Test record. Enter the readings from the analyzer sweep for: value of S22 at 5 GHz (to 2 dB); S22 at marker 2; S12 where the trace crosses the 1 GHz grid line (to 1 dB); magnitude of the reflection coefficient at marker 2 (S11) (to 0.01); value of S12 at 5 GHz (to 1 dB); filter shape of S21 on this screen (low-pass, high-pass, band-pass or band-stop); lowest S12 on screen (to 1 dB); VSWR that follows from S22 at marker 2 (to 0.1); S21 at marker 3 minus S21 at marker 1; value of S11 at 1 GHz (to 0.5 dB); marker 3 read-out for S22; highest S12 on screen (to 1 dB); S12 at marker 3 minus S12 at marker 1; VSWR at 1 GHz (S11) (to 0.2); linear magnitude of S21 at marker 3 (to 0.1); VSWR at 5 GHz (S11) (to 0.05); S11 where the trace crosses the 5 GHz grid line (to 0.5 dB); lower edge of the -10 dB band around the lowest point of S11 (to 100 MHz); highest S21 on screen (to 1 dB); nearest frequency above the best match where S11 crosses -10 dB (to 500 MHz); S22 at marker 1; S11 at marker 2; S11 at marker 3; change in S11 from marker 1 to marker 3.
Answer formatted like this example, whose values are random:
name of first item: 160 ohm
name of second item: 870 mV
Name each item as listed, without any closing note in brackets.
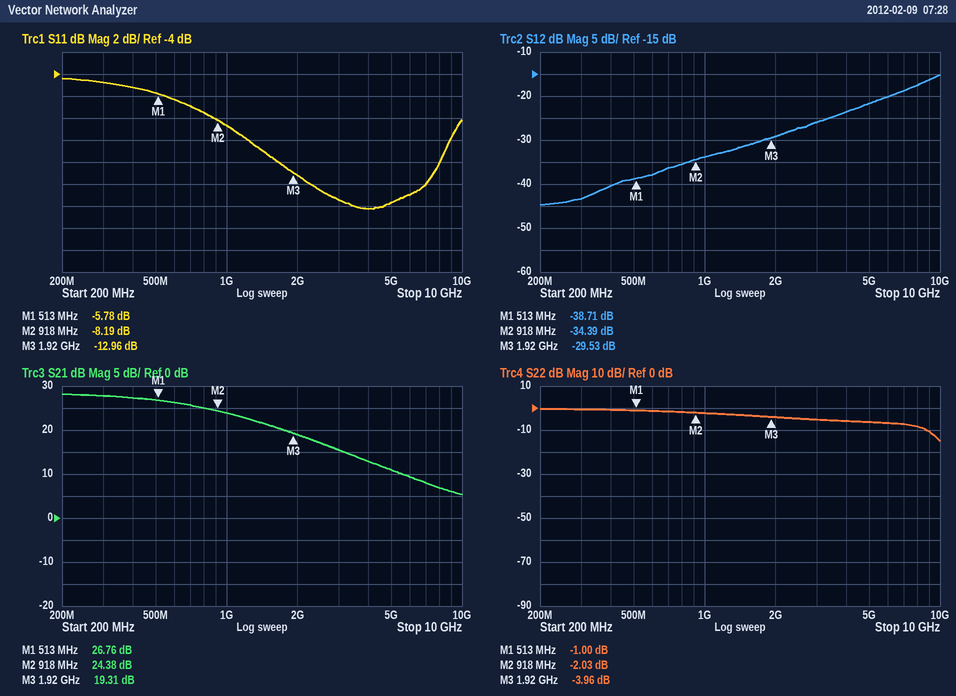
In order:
value of S22 at 5 GHz: -6 dB
S22 at marker 2: -2.03 dB
S12 where the trace crosses the 1 GHz grid line: -34 dB
magnitude of the reflection coefficient at marker 2 (S11): 0.39
value of S12 at 5 GHz: -22 dB
filter shape of S21 on this screen: low-pass
lowest S12 on screen: -45 dB
VSWR that follows from S22 at marker 2: 8.6
S21 at marker 3 minus S21 at marker 1: -7.45 dB
value of S11 at 1 GHz: -8.5 dB
marker 3 read-out for S22: -3.96 dB
highest S12 on screen: -15 dB
S12 at marker 3 minus S12 at marker 1: 9.18 dB
VSWR at 1 GHz (S11): 2.2
linear magnitude of S21 at marker 3: 9.2
VSWR at 5 GHz (S11): 1.40
S11 where the trace crosses the 5 GHz grid line: -15.5 dB
lower edge of the -10 dB band around the lowest point of S11: 1.2 GHz
highest S21 on screen: 28 dB
nearest frequency above the best match where S11 crosses -10 dB: 9.0 GHz
S22 at marker 1: -1.00 dB
S11 at marker 2: -8.19 dB
S11 at marker 3: -12.96 dB
change in S11 from marker 1 to marker 3: -7.18 dB
